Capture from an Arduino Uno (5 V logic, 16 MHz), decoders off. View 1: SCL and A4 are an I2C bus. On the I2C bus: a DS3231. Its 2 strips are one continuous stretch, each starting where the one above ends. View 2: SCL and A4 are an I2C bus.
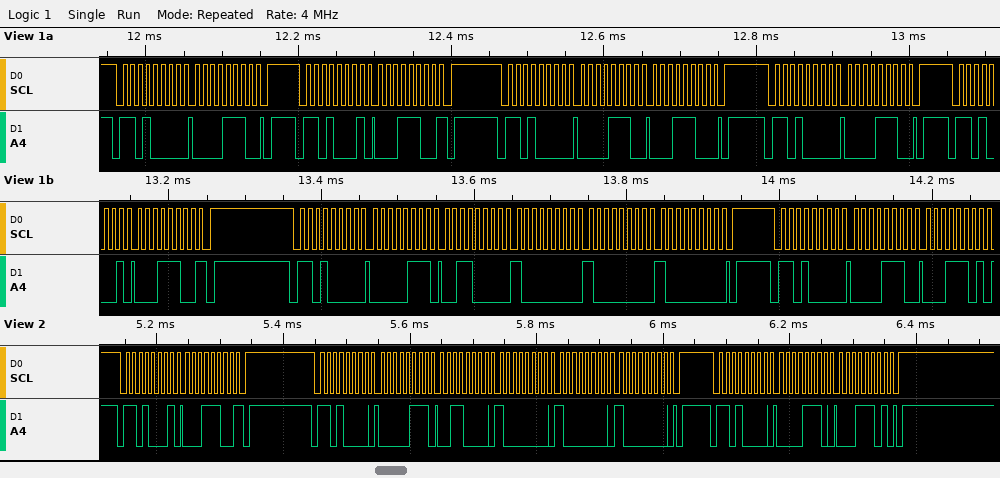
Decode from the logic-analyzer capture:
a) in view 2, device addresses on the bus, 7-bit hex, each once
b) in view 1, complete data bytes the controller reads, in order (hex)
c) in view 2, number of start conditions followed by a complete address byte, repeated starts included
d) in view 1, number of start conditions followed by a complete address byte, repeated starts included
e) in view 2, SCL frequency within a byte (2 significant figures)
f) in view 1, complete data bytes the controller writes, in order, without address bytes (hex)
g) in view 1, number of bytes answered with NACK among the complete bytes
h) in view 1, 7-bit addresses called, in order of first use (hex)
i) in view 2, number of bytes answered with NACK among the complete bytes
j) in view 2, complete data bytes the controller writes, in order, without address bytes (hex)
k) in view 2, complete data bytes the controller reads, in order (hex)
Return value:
0x68
1C 1C
3
7
100 kHz
0E 0E 1C 0E 07 30 80 80 80 0E 1D
2
0x68
1
07 30 80 80 80 0E 1D
1C
